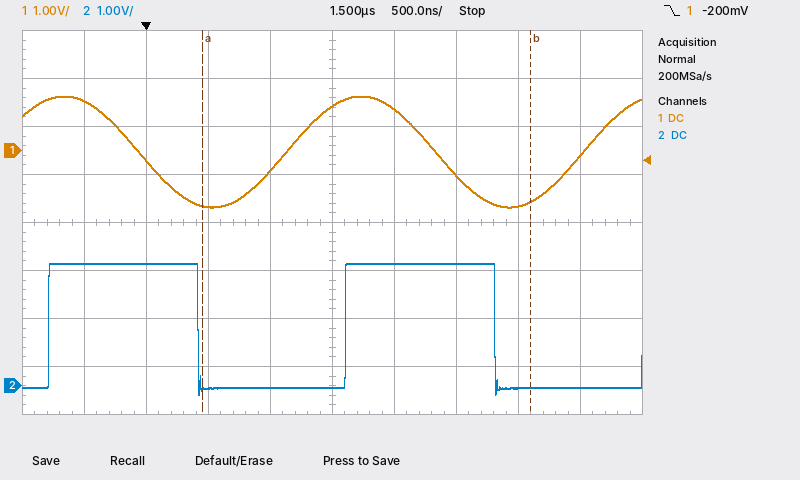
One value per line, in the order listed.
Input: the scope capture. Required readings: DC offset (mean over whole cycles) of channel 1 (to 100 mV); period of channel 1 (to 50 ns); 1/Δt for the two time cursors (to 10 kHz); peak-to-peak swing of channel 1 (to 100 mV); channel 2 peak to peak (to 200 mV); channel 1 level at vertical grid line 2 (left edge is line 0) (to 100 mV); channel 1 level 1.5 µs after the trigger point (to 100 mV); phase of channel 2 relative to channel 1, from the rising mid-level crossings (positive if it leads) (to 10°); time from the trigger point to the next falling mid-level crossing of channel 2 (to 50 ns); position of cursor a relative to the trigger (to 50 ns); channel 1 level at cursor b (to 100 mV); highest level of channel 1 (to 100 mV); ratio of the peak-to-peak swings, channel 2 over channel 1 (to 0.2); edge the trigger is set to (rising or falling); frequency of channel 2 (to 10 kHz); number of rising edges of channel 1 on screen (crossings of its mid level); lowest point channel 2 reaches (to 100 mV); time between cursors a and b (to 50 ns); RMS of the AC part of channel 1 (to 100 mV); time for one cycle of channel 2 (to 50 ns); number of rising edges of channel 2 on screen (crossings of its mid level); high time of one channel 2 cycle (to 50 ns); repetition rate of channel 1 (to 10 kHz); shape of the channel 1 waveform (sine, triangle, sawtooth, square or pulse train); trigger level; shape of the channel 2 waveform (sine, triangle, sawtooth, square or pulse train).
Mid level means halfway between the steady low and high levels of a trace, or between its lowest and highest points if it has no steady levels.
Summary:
0.0 V
2.40 µs
380 kHz
2.3 V
2.8 V
-200 mV
900 mV
-70°
400 ns
+450 ns
-1.1 V
1.1 V
1.2
falling
420 kHz
2
-200 mV
2.65 µs
800 mV
2.40 µs
2
1.20 µs
420 kHz
sine
-200 mV
square
